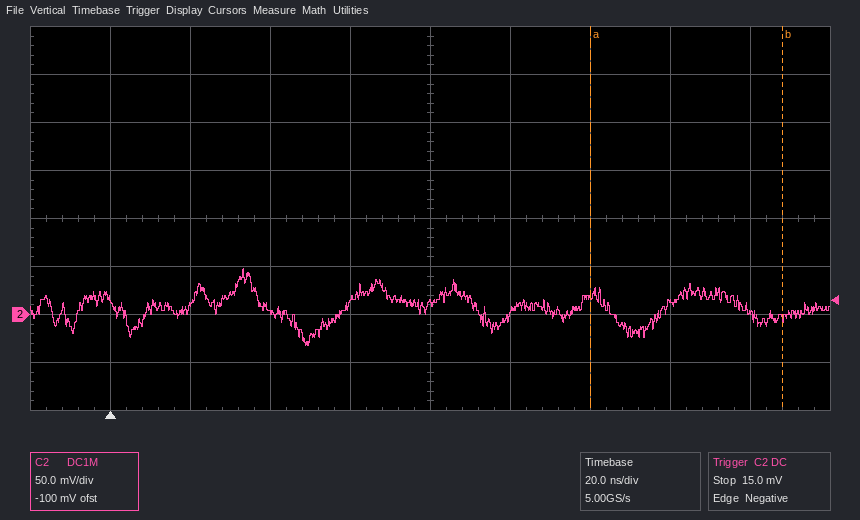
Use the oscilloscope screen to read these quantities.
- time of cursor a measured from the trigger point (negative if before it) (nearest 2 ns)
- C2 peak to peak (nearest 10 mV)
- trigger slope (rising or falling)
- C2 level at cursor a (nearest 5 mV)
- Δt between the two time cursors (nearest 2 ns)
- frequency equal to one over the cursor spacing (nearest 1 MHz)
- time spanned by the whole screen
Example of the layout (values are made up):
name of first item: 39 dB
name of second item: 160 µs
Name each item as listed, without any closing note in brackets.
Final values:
time of cursor a measured from the trigger point (negative if before it): +120 ns
C2 peak to peak: 80 mV
trigger slope: falling
C2 level at cursor a: 20 mV
Δt between the two time cursors: 48 ns
frequency equal to one over the cursor spacing: 21 MHz
time spanned by the whole screen: 200 ns
